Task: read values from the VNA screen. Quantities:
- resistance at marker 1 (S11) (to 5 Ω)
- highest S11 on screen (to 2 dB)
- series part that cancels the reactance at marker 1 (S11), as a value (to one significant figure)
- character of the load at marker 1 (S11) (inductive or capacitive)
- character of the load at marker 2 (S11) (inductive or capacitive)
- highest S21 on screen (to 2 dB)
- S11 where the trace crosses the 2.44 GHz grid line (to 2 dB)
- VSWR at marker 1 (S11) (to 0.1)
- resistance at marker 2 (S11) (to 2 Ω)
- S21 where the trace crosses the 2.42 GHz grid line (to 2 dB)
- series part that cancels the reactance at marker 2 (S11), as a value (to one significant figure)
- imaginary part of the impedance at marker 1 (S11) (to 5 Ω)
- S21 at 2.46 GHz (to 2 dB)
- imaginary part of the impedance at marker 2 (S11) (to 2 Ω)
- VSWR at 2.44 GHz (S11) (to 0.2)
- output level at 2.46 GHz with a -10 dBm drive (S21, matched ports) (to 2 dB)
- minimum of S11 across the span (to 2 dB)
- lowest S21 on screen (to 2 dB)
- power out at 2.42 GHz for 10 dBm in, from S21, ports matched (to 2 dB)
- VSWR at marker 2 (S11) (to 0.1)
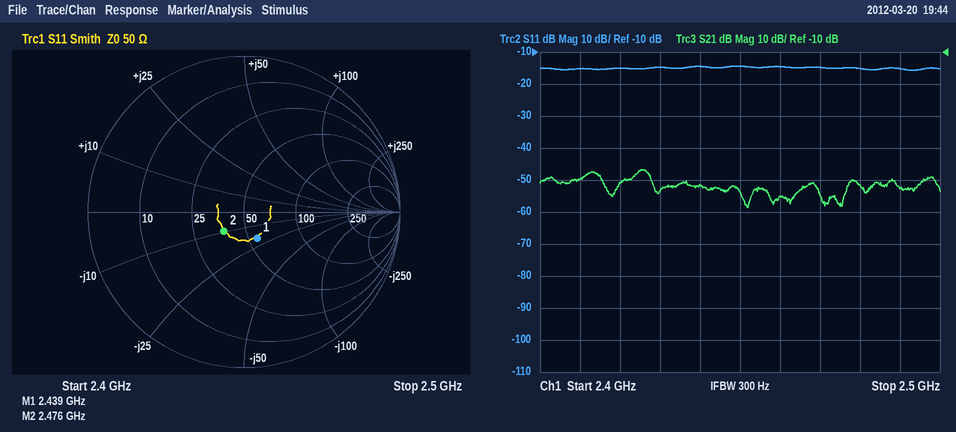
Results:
55 Ω
-14 dB
1 nH
capacitive
capacitive
-46 dB
-14 dB
1.5
38 Ω
-50 dB
600 pH
-20 Ω
-56 dB
-10 Ω
1.4
-66 dBm
-16 dB
-58 dB
-40 dBm
1.4
